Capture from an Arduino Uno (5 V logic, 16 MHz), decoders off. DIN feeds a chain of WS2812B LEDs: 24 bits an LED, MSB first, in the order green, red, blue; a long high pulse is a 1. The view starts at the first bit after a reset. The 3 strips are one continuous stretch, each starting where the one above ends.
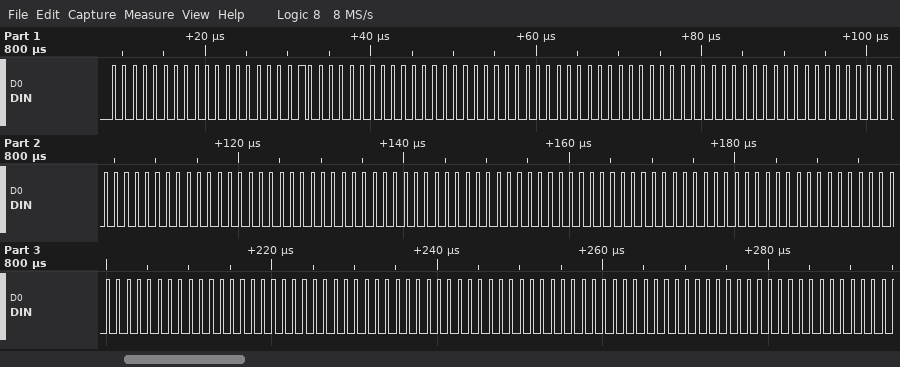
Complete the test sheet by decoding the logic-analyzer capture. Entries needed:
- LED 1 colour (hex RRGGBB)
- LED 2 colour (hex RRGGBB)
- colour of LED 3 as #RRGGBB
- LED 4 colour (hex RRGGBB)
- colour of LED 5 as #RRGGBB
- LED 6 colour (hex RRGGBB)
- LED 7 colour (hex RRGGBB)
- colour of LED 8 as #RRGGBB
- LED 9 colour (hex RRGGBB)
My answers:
#000020
#000000
#000000
#000000
#000000
#000000
#000000
#000000
#000000
